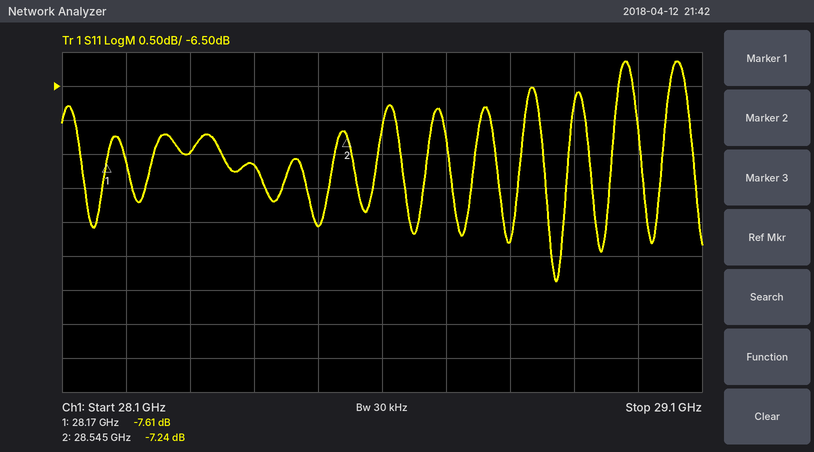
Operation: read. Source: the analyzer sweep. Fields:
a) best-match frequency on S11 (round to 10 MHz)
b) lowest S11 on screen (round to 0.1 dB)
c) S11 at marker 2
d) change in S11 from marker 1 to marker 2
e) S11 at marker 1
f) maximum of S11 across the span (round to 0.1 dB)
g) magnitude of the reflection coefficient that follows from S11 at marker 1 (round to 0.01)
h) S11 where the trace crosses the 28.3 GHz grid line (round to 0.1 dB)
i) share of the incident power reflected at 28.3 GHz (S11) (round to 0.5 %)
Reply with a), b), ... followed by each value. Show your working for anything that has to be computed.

a) 28.87 GHz
b) -9.4 dB
c) -7.24 dB
d) -7.24 − (-7.61) = 0.37 dB
e) -7.61 dB
f) -6.1 dB
g) 10^(-7.61/20) ≈ 0.42
h) -7.5 dB
i) 10^(-7.5/10) ≈ 17.8 %, so 18.0 % to the nearest 0.5 %
